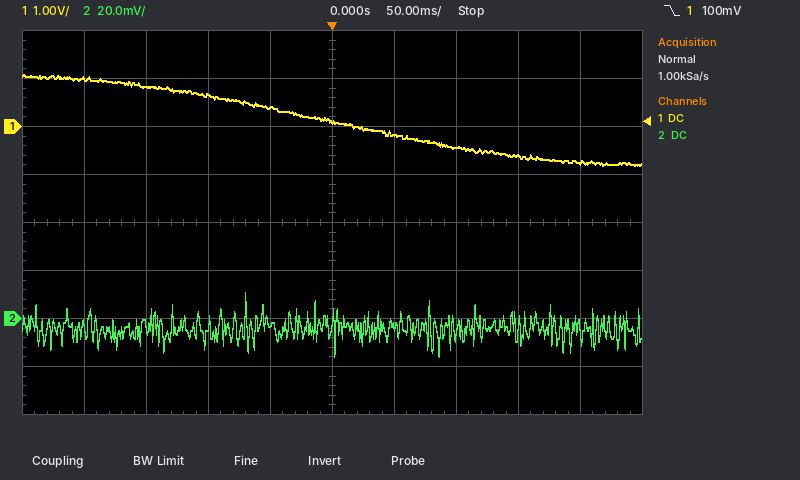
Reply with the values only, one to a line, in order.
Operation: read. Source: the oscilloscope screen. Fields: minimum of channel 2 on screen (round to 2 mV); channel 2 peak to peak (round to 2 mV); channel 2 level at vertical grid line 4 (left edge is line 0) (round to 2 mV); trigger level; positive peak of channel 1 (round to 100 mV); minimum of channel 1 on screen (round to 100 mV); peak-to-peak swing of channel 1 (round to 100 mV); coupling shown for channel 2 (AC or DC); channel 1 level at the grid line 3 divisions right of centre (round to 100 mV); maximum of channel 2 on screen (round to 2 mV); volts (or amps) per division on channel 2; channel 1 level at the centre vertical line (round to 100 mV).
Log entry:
-16 mV
26 mV
-2 mV
100 mV
1.1 V
-800 mV
1.9 V
DC
-600 mV
10 mV
20 mV
100 mV
